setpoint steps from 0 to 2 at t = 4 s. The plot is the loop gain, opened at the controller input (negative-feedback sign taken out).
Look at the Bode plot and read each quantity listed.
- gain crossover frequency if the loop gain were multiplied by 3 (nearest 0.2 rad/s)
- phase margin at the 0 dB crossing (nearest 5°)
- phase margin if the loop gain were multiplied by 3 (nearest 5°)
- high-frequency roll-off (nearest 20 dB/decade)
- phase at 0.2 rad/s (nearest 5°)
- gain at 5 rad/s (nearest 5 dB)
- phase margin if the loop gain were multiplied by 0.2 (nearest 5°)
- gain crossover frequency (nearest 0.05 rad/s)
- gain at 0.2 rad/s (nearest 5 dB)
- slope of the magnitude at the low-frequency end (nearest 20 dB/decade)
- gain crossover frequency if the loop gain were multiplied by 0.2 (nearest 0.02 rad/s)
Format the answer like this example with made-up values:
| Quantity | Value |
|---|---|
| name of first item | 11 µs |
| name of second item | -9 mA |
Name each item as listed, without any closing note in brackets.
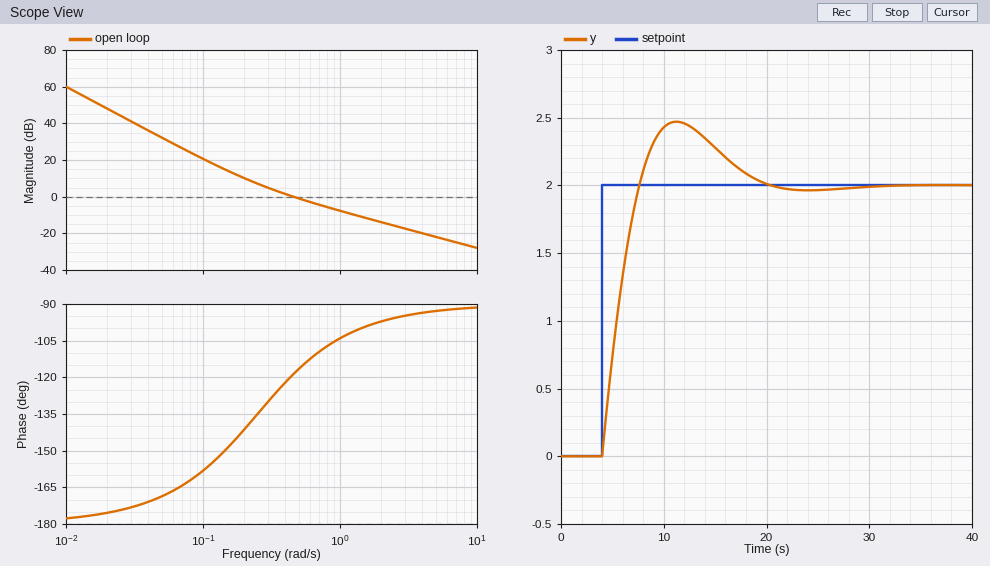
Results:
| Quantity | Value |
|---|---|
| gain crossover frequency if the loop gain were multiplied by 3 | 1.2 rad/s |
| phase margin at the 0 dB crossing | 60° |
| phase margin if the loop gain were multiplied by 3 | 80° |
| high-frequency roll-off | -20 dB/decade |
| phase at 0.2 rad/s | -140° |
| gain at 5 rad/s | -20 dB |
| phase margin if the loop gain were multiplied by 0.2 | 30° |
| gain crossover frequency | 0.45 rad/s |
| gain at 0.2 rad/s | 10 dB |
| slope of the magnitude at the low-frequency end | -40 dB/decade |
| gain crossover frequency if the loop gain were multiplied by 0.2 | 0.16 rad/s |
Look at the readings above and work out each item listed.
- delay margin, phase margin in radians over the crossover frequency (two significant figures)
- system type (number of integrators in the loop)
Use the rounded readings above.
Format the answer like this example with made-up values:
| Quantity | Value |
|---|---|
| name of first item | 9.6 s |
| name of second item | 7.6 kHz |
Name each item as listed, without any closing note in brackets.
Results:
| Quantity | Value |
|---|---|
| delay margin, phase margin in radians over the crossover frequency | 2.3 s |
| system type | 2 |
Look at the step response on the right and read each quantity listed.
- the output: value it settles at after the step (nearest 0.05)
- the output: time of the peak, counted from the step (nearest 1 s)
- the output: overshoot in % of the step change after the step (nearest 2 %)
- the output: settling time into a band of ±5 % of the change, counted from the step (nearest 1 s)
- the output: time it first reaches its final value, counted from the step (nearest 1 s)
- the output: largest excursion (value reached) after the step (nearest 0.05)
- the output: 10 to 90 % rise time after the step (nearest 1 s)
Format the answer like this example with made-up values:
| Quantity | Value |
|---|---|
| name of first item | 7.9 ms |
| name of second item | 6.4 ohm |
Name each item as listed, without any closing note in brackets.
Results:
| Quantity | Value |
|---|---|
| the output: value it settles at after the step | 2.00 |
| the output: time of the peak, counted from the step | 7 s |
| the output: overshoot in % of the step change after the step | 24 % |
| the output: settling time into a band of ±5 % of the change, counted from the step | 14 s |
| the output: time it first reaches its final value, counted from the step | 4 s |
| the output: largest excursion (value reached) after the step | 2.45 |
| the output: 10 to 90 % rise time after the step | 3 s |
